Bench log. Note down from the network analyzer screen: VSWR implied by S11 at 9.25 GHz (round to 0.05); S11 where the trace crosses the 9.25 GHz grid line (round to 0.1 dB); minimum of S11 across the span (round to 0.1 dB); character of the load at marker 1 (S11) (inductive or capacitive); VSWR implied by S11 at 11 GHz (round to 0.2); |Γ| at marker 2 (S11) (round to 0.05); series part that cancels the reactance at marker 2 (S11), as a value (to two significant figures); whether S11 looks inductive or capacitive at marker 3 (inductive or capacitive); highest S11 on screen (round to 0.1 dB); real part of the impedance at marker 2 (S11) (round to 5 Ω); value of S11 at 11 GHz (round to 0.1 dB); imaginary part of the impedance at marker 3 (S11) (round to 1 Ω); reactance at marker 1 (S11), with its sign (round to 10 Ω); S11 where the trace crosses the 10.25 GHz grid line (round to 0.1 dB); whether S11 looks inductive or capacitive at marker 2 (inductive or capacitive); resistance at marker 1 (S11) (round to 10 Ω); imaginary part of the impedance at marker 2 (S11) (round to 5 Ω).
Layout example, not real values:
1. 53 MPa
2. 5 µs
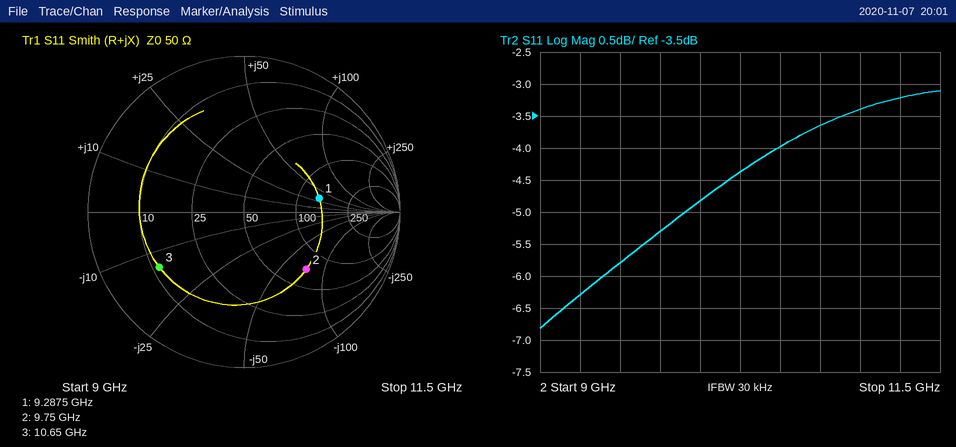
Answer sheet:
1. 2.90
2. -6.3 dB
3. -6.8 dB
4. inductive
5. 5.2
6. 0.55
7. 1.2 nH
8. capacitive
9. -3.1 dB
10. 70 Ω
11. -3.4 dB
12. -14 Ω
13. +30 Ω
14. -4.4 dB
15. capacitive
16. 140 Ω
17. -75 Ω
